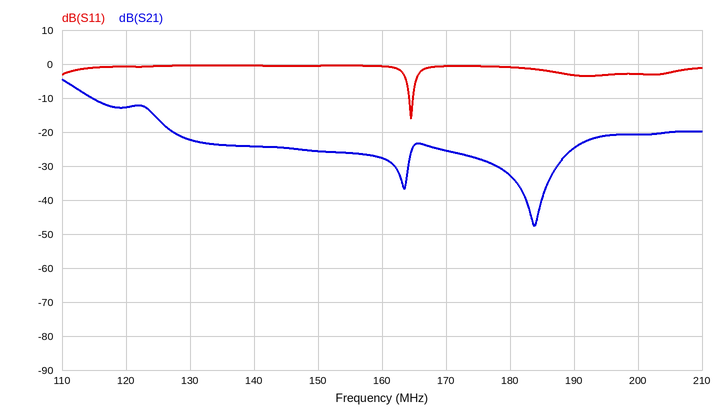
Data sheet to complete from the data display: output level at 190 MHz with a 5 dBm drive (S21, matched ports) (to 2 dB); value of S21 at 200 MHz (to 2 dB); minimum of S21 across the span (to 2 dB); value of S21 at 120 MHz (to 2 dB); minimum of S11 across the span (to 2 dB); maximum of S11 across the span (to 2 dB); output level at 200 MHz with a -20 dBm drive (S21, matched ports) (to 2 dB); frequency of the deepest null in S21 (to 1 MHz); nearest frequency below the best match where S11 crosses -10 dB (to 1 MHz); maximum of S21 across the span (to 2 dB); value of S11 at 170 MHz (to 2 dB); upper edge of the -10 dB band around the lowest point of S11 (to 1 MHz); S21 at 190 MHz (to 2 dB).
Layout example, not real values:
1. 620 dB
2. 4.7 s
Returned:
1. -20 dBm
2. -20 dB
3. -48 dB
4. -12 dB
5. -16 dB
6. 0 dB
7. -40 dBm
8. 184 MHz
9. 164 MHz
10. -4 dB
11. 0 dB
12. 165 MHz
13. -24 dB
